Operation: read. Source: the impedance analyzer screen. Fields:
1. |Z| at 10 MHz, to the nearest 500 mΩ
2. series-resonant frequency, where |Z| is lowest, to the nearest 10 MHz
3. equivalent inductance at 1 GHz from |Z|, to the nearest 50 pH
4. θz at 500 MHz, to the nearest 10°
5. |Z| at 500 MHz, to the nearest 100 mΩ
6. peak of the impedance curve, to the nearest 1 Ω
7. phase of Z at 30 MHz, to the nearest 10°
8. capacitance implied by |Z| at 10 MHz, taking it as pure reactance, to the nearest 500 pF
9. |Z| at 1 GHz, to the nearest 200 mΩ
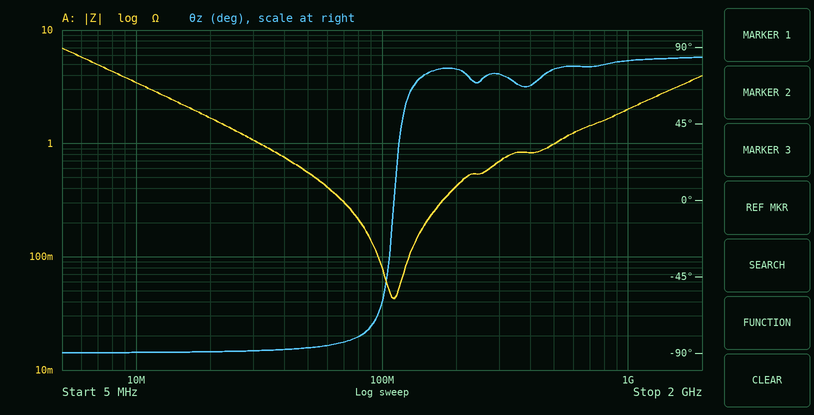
3.5 Ω
110 MHz
300 pH
80°
1.0 Ω
7 Ω
-90°
4.5 nF
2.0 Ω
